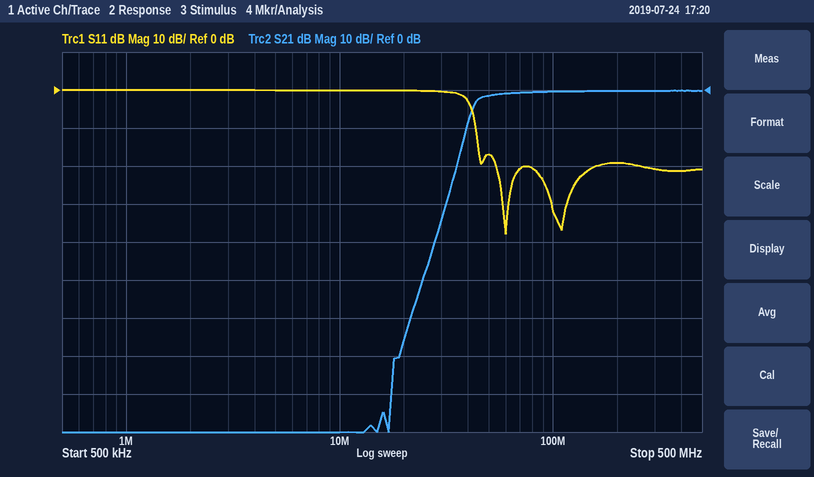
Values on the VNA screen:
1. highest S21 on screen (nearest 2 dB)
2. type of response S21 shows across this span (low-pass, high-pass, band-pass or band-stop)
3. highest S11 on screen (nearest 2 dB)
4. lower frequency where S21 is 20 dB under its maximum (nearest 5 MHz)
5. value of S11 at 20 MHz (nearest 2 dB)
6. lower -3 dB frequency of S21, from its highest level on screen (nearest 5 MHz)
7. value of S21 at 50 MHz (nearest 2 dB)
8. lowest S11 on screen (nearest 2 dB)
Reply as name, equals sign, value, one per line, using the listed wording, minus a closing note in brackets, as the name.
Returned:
highest S21 on screen = 0 dB
type of response S21 shows across this span = high-pass
highest S11 on screen = 0 dB
lower frequency where S21 is 20 dB under its maximum = 35 MHz
value of S11 at 20 MHz = 0 dB
lower -3 dB frequency of S21, from its highest level on screen = 45 MHz
value of S21 at 50 MHz = -2 dB
lowest S11 on screen = -38 dB
